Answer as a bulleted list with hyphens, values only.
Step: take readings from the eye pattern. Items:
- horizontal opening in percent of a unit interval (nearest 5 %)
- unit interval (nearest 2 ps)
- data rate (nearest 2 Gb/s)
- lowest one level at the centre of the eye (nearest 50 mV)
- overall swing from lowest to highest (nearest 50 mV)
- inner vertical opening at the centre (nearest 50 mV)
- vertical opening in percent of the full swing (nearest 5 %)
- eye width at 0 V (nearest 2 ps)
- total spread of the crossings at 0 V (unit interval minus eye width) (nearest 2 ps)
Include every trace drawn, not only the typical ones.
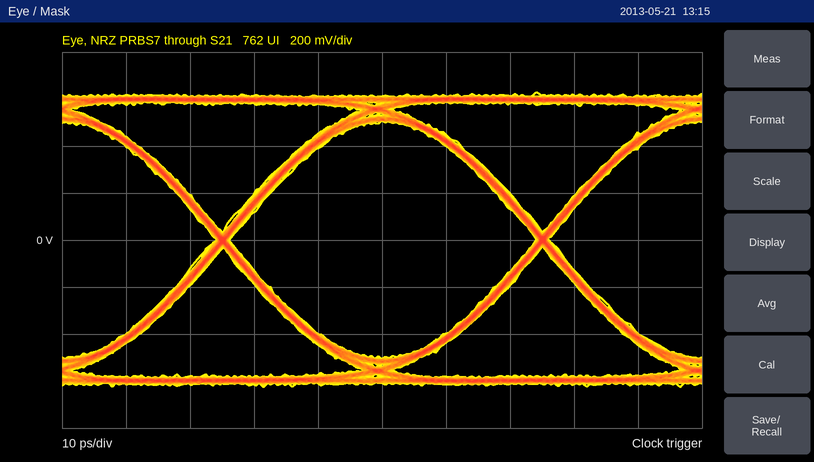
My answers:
- 95 %
- 50 ps
- 20 Gb/s
- 500 mV
- 1.25 V
- 1.00 V
- 80 %
- 48 ps
- 2 ps
